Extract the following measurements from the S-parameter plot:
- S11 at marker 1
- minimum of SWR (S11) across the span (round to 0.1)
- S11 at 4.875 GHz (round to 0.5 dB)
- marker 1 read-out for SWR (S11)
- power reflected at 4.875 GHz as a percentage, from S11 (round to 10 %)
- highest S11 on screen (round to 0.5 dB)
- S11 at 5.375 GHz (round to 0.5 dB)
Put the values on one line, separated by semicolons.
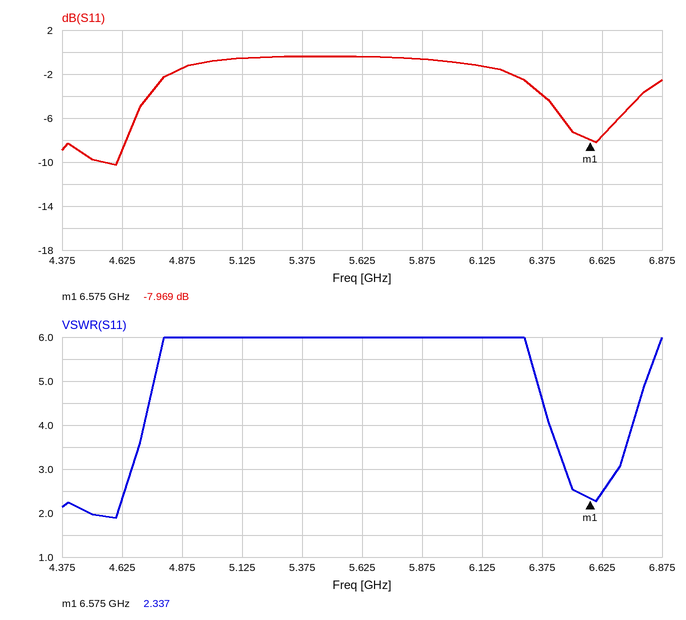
-7.969 dB; 1.9; -1.5 dB; 2.337; 70 %; -0.5 dB; -0.5 dB
